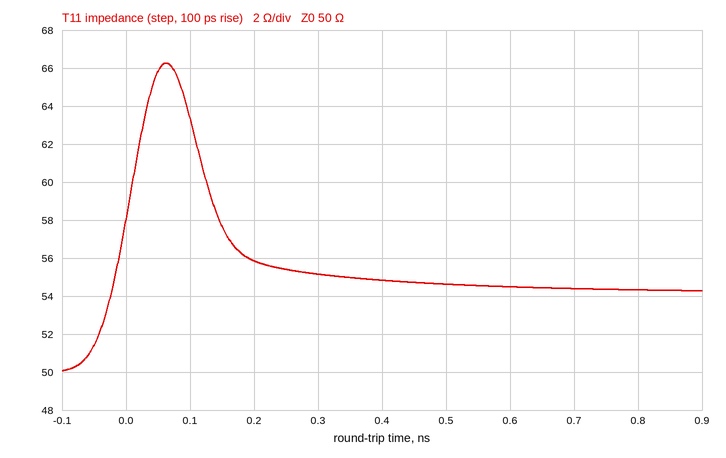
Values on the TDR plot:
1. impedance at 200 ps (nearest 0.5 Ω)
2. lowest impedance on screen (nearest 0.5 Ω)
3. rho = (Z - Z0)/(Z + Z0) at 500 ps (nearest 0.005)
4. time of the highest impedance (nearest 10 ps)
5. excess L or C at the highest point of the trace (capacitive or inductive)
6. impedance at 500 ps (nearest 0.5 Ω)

56.0 Ω
50.0 Ω
+0.045
60 ps
inductive
54.5 Ω
